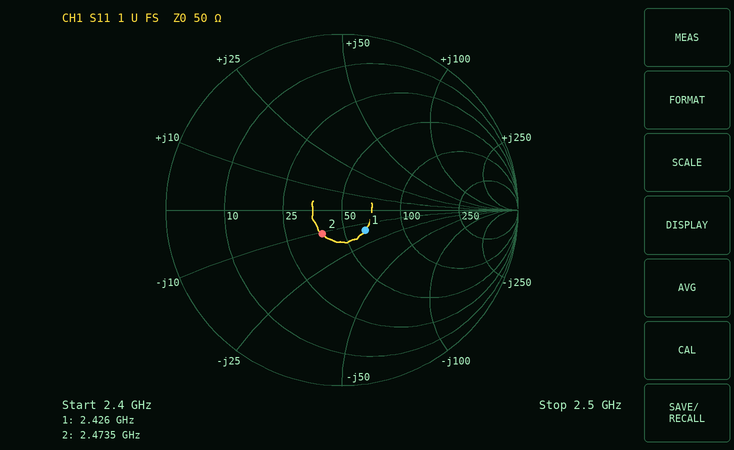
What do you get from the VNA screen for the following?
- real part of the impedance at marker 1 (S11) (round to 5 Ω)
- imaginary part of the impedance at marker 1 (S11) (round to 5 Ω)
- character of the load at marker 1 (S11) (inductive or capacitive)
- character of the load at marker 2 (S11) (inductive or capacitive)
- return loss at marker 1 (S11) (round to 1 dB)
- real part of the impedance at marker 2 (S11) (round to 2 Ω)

65 Ω
-15 Ω
capacitive
capacitive
15 dB
38 Ω
